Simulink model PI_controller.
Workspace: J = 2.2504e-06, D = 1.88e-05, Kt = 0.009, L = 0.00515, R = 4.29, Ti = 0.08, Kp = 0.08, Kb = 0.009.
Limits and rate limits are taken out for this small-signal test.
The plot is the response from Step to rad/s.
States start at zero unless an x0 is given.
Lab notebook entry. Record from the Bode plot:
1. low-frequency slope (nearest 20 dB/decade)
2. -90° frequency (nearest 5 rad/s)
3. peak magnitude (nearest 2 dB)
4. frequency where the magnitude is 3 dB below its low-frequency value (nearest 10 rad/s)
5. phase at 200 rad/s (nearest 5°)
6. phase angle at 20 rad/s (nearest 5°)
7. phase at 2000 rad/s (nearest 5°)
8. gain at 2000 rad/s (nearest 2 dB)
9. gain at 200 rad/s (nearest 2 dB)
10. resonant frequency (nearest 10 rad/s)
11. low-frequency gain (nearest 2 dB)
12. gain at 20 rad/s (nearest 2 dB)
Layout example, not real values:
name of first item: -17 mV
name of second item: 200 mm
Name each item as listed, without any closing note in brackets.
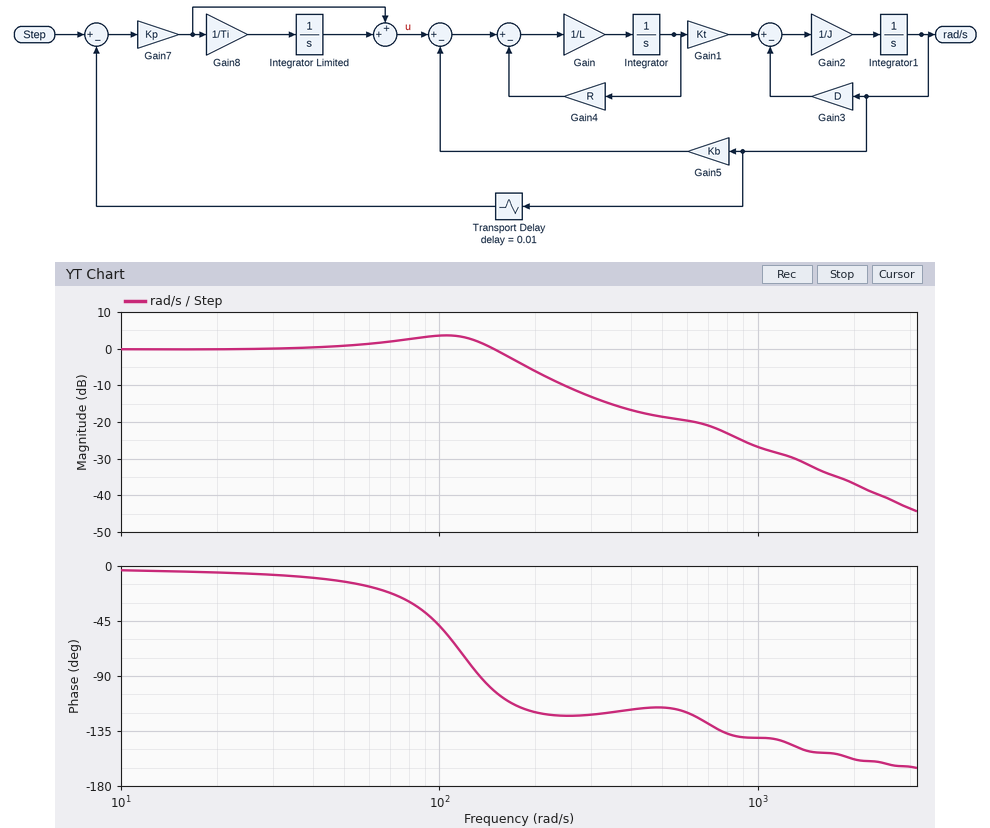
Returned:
low-frequency slope: 0 dB/decade
-90° frequency: 135 rad/s
peak magnitude: 4 dB
frequency where the magnitude is 3 dB below its low-frequency value: 170 rad/s
phase at 200 rad/s: -120°
phase angle at 20 rad/s: -5°
phase at 2000 rad/s: -160°
gain at 2000 rad/s: -36 dB
gain at 200 rad/s: -6 dB
resonant frequency: 100 rad/s
low-frequency gain: 0 dB
gain at 20 rad/s: 0 dB
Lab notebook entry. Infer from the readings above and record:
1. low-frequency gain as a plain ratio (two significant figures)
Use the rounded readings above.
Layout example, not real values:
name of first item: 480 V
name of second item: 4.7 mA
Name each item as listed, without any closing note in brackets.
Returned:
low-frequency gain as a plain ratio: 1.0
